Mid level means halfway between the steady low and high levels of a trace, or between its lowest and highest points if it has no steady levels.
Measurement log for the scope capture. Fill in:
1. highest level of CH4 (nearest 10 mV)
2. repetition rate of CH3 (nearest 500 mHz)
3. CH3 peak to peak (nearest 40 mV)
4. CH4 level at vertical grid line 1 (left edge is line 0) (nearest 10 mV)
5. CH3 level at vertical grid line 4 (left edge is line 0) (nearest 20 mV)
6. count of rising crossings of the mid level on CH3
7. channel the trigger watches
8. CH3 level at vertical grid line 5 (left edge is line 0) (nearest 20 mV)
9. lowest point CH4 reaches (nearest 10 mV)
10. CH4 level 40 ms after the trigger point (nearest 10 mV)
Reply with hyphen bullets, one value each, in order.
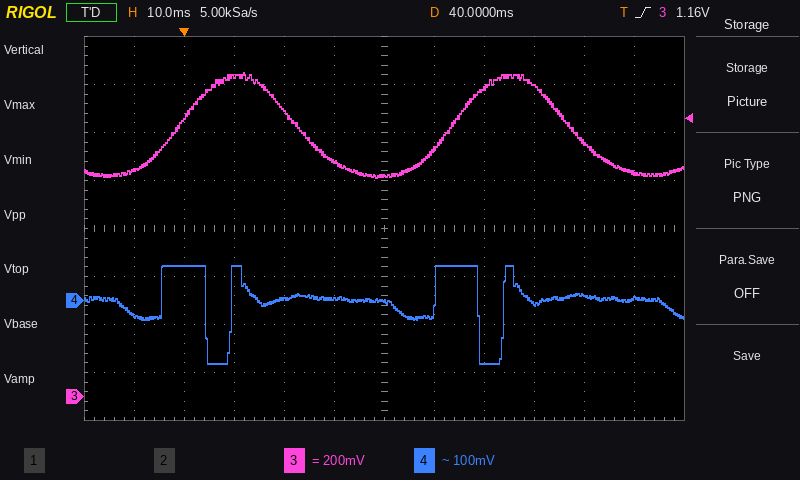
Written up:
- 70 mV
- 18.5 Hz
- 440 mV
- -30 mV
- 1.20 V
- 2
- CH3
- 980 mV
- -130 mV
- 0 mV
